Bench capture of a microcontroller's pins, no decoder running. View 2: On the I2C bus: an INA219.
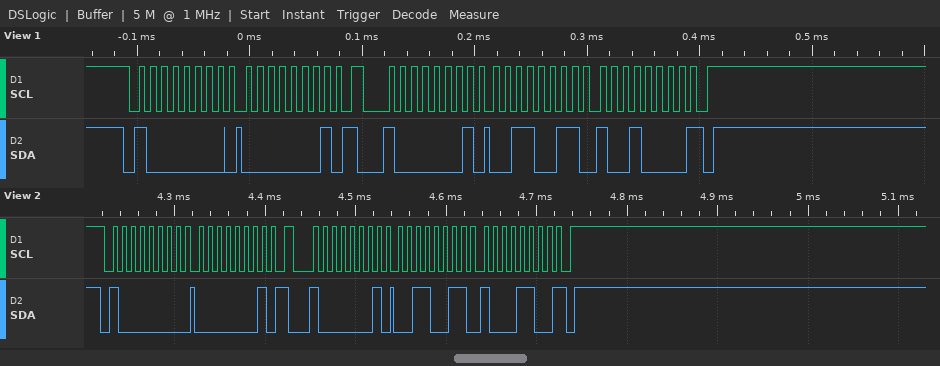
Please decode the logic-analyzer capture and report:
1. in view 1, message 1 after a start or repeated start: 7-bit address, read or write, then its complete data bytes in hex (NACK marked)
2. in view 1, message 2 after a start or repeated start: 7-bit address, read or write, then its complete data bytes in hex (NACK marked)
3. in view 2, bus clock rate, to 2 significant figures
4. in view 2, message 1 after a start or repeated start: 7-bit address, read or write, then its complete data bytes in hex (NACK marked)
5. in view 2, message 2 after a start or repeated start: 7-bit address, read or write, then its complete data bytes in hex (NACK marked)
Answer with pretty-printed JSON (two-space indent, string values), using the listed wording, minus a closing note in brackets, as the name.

{
  "in view 1, message 1 after a start or repeated start: 7-bit address, read or write, then its complete data bytes in hex": "0x40 write: 01",
  "in view 1, message 2 after a start or repeated start: 7-bit address, read or write, then its complete data bytes in hex": "0x40 read: 33 90 NACK",
  "in view 2, bus clock rate, to 2 significant figures": "100 kHz",
  "in view 2, message 1 after a start or repeated start: 7-bit address, read or write, then its complete data bytes in hex": "0x40 write: 01",
  "in view 2, message 2 after a start or repeated start: 7-bit address, read or write, then its complete data bytes in hex": "0x40 read: 33 8C NACK"
}
